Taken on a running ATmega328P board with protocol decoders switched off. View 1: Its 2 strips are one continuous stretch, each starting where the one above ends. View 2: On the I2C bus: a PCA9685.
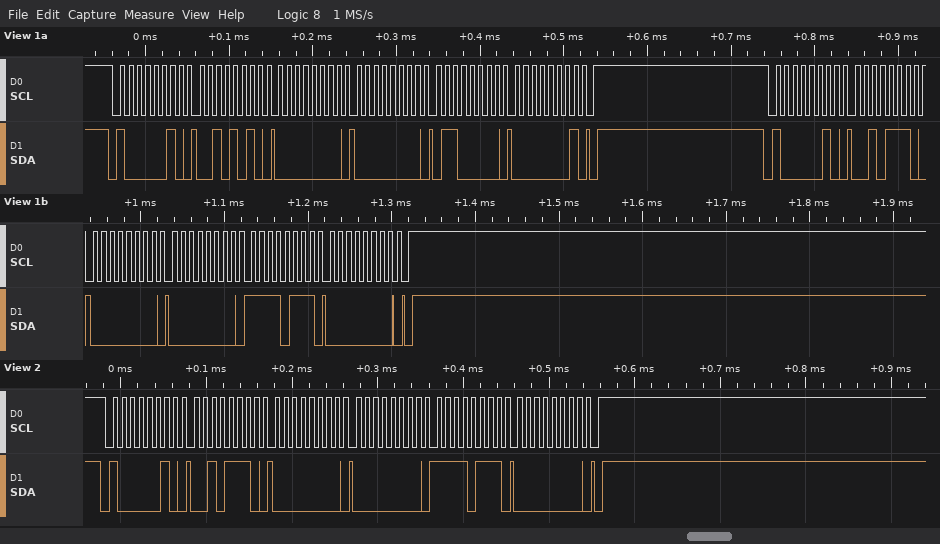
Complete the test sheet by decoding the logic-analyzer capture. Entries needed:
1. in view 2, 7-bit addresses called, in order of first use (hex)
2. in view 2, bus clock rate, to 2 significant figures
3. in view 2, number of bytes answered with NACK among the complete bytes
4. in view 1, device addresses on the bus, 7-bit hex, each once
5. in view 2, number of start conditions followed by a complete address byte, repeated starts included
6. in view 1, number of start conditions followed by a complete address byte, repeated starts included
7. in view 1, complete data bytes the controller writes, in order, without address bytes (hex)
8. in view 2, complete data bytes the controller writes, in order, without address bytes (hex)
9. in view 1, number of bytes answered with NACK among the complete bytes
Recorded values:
0x41
100 kHz
0
0x41
1
2
2A 00 00 60 01 2E 00 00 F7 00
2E 00 00 F7 00
0
